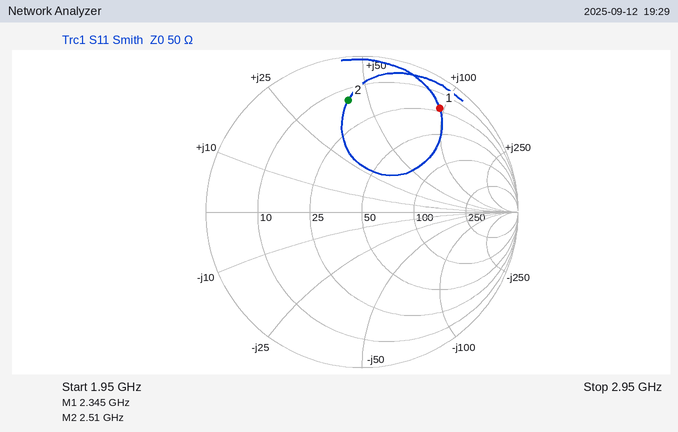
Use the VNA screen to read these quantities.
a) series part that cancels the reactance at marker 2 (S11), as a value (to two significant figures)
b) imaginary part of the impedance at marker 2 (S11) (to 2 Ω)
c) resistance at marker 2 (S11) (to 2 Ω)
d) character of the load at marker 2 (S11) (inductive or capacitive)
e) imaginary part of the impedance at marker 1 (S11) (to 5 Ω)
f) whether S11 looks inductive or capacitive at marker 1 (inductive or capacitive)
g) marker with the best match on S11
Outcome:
1.5 pF
+42 Ω
14 Ω
inductive
+95 Ω
inductive
marker 2
